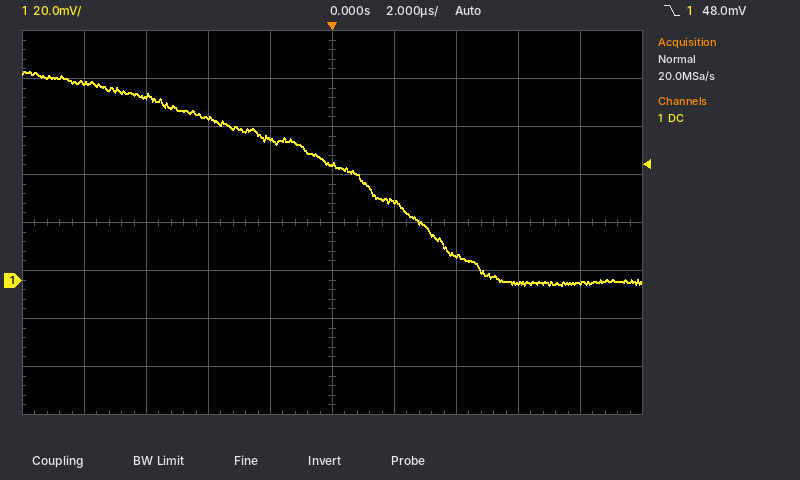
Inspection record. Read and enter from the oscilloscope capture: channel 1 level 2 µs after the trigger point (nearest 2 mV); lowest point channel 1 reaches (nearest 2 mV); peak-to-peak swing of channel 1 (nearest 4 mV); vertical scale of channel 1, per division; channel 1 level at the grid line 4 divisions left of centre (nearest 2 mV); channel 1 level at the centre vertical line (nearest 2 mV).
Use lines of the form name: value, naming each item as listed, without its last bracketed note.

channel 1 level 2 µs after the trigger point: 32 mV
lowest point channel 1 reaches: -2 mV
peak-to-peak swing of channel 1: 88 mV
vertical scale of channel 1, per division: 20 mV
channel 1 level at the grid line 4 divisions left of centre: 82 mV
channel 1 level at the centre vertical line: 48 mV
